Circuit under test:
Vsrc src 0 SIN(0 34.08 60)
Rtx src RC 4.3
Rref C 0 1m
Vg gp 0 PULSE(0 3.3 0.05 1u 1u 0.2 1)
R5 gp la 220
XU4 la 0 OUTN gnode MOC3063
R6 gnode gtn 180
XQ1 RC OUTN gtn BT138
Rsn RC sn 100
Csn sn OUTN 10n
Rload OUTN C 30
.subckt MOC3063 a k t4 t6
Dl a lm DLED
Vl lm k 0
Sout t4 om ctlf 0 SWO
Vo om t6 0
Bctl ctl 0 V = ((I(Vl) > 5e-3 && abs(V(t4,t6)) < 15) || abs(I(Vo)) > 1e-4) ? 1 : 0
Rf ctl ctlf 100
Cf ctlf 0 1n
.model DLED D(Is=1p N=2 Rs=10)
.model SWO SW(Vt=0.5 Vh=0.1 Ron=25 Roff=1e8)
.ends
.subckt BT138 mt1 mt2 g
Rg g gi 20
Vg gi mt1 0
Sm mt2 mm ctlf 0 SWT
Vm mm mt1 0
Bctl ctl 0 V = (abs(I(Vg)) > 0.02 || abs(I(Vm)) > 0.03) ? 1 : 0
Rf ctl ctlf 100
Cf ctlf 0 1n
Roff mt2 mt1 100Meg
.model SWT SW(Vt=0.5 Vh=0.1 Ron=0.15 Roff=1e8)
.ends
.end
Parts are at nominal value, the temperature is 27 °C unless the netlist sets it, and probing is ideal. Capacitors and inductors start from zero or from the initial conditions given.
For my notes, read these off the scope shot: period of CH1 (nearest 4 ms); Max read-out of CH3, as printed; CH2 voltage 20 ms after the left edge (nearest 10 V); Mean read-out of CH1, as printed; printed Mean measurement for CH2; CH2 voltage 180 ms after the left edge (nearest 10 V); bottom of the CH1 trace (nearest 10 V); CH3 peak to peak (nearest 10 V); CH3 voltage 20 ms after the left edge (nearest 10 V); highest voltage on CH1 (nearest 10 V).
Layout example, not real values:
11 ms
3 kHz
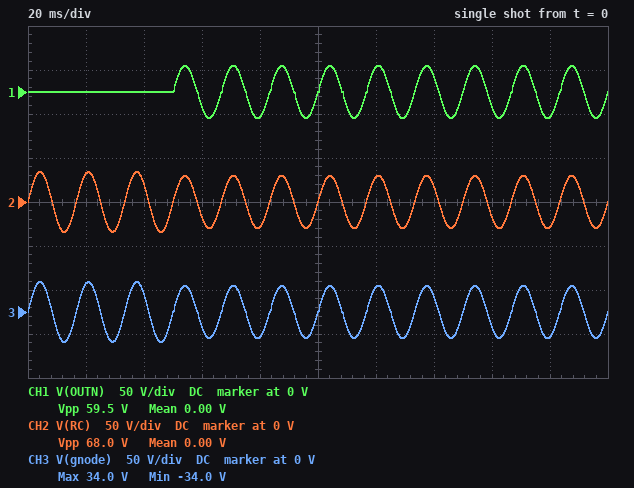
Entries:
16 ms
34.0 V
30 V
0.00 V
0.00 V
-30 V
-30 V
70 V
30 V
30 V
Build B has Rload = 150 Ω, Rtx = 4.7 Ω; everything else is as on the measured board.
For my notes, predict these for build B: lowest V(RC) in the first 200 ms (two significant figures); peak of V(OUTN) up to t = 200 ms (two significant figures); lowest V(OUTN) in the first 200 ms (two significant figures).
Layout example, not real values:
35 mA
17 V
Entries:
-34 V
33 V
-33 V
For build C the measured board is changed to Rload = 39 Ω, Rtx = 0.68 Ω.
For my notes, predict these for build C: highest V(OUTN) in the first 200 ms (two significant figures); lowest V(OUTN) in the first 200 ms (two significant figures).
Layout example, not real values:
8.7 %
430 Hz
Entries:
33 V
-33 V
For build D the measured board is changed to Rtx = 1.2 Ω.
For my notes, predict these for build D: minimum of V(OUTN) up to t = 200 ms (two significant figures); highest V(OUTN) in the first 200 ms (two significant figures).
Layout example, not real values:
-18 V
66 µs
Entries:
-33 V
33 V
